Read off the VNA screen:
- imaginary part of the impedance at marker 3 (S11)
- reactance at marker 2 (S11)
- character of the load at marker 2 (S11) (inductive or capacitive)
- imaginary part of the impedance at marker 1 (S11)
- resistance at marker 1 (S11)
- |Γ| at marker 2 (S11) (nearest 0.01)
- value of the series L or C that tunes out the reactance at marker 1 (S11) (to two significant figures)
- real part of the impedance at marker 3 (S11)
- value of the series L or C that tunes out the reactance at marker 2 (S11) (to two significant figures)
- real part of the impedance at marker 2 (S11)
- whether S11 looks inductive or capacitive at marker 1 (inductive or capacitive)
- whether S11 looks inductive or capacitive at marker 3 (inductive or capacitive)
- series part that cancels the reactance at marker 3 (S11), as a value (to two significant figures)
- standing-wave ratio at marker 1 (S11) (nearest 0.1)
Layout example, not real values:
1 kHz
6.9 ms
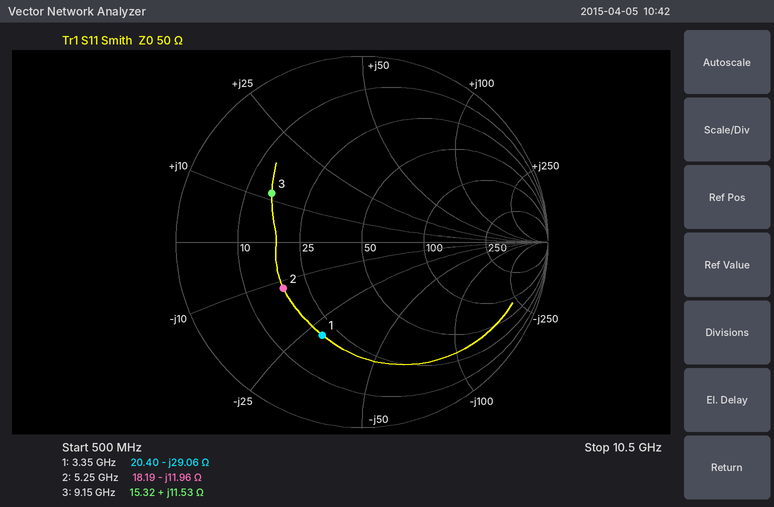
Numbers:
+11.53 Ω
-11.96 Ω
capacitive
-29.06 Ω
20.40 Ω
0.49
1.4 nH
15.32 Ω
360 pH
18.19 Ω
capacitive
inductive
1.5 pF
3.4
